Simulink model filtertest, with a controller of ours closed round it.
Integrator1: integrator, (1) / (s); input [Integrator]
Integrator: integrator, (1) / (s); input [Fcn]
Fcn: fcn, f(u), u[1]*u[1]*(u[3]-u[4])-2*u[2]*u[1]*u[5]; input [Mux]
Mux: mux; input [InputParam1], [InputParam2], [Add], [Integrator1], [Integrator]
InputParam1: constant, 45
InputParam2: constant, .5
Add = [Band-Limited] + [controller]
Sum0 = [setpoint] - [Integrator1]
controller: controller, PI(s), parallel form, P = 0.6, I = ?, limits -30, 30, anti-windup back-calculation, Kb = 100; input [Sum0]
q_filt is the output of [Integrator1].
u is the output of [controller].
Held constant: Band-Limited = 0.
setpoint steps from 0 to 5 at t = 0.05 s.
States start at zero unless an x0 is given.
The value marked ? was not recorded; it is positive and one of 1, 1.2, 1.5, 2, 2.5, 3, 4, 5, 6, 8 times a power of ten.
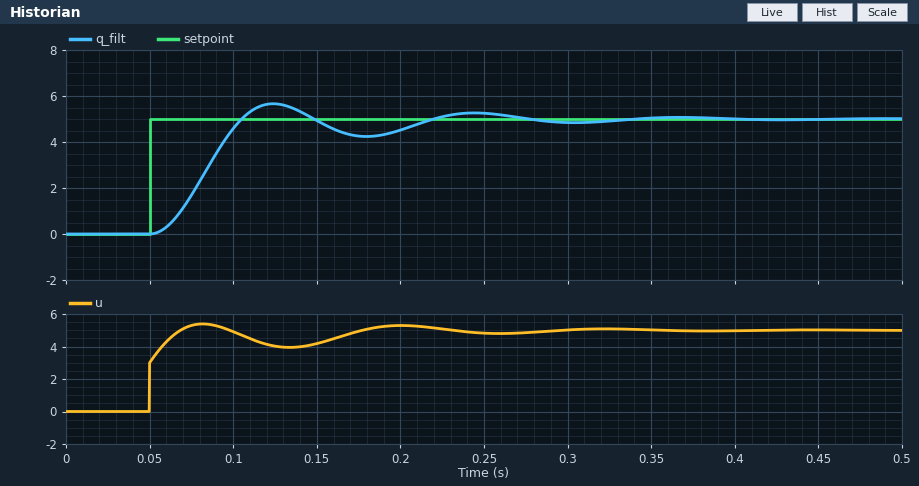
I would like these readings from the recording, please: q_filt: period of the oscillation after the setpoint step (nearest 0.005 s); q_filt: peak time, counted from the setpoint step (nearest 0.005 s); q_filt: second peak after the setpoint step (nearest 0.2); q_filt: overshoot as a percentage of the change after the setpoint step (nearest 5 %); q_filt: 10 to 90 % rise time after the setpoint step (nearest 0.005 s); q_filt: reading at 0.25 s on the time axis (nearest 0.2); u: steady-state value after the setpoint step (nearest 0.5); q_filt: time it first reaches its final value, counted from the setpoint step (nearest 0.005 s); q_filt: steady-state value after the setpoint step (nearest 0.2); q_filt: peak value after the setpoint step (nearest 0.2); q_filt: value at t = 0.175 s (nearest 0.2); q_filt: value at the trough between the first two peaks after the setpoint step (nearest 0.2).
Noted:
0.120 s
0.075 s
5.2
15 %
0.035 s
5.2
5.0
0.055 s
5.0
5.6
4.2
4.2
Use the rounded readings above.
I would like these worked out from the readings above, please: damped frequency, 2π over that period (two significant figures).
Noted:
52 rad/s
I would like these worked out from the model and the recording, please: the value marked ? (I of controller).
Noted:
30
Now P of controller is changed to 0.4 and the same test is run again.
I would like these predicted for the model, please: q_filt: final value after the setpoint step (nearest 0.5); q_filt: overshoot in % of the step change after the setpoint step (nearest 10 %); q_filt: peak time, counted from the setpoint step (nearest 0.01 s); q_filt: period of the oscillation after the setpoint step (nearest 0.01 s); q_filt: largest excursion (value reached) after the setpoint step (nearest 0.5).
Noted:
5.0
20 %
0.08 s
0.13 s
6.0
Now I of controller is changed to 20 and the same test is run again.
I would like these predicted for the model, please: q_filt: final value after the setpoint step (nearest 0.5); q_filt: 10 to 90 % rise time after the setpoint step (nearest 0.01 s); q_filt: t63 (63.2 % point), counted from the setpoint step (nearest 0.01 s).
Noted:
5.0
0.05 s
0.04 s
